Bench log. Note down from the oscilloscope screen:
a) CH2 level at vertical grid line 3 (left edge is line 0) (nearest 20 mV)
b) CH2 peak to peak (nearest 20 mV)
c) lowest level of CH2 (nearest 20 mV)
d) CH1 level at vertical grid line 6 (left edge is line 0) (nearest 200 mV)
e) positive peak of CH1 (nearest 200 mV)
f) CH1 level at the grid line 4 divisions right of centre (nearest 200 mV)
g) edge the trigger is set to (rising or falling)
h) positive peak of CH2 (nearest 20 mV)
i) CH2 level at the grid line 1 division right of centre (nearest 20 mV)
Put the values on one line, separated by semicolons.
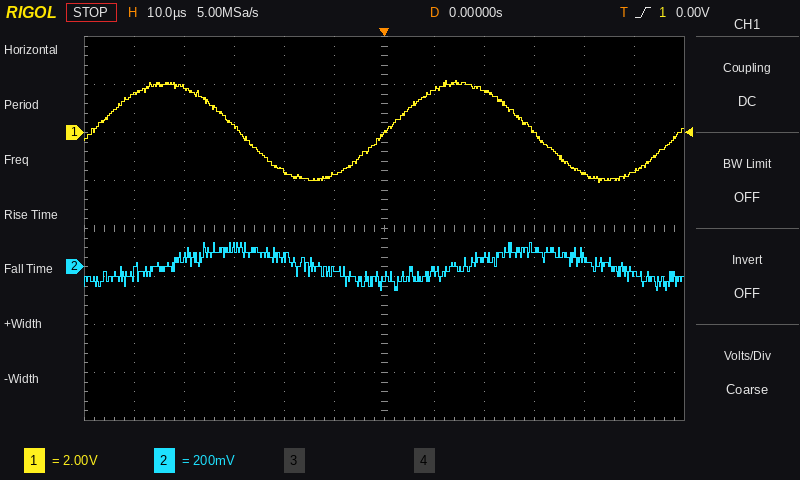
80 mV; 200 mV; -100 mV; 0.0 V; 2.2 V; -1.8 V; rising; 100 mV; -20 mV
